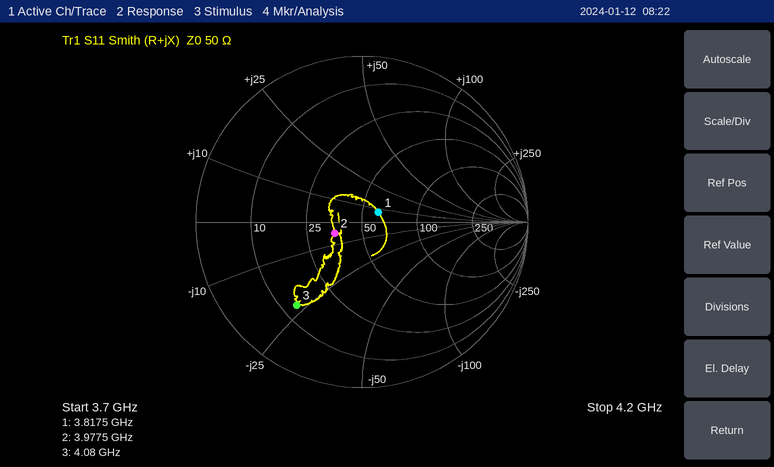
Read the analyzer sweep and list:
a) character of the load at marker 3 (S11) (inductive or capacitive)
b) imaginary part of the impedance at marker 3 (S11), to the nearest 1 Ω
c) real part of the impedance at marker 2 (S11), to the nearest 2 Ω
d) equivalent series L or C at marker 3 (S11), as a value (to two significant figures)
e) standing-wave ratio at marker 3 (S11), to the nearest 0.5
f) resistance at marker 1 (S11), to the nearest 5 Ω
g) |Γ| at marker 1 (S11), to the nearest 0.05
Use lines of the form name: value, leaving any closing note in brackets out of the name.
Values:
character of the load at marker 3 (S11): capacitive
imaginary part of the impedance at marker 3 (S11), to the nearest 1 Ω: -23 Ω
real part of the impedance at marker 2 (S11), to the nearest 2 Ω: 36 Ω
equivalent series L or C at marker 3 (S11), as a value: 1.7 pF
standing-wave ratio at marker 3 (S11), to the nearest 0.5: 4.5
resistance at marker 1 (S11), to the nearest 5 Ω: 60 Ω
|Γ| at marker 1 (S11), to the nearest 0.05: 0.10
